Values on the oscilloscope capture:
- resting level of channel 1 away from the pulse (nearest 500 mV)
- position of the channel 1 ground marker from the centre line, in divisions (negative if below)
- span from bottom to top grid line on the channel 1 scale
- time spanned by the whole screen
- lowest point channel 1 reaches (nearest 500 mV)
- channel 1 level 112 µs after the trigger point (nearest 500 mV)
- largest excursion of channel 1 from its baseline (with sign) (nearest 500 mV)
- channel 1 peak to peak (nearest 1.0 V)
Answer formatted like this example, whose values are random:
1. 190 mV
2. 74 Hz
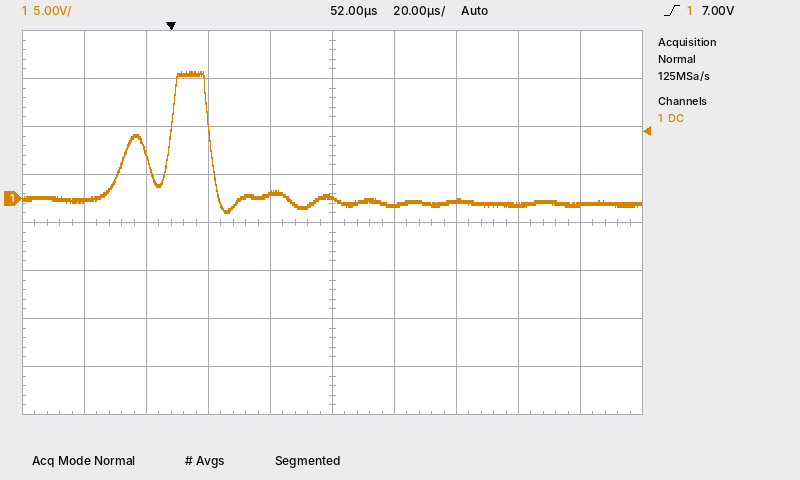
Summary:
1. -500 mV
2. +0.5 div
3. 40 V
4. 200 µs
5. -1.5 V
6. -500 mV
7. +13.5 V
8. 15.0 V
